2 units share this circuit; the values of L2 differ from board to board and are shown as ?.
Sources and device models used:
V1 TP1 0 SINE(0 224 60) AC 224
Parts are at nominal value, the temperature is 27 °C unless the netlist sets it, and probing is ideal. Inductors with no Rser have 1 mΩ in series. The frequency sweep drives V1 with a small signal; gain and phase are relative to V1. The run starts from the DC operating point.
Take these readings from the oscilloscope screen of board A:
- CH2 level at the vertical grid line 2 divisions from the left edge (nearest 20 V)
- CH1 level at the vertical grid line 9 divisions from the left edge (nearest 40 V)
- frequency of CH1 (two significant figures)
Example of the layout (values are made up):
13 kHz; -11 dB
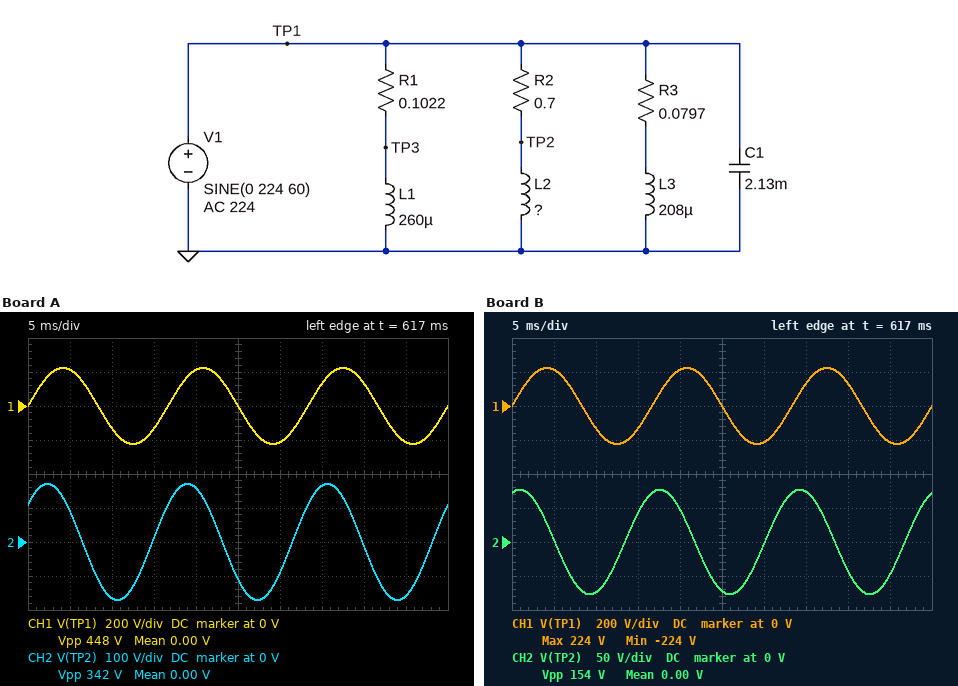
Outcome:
-160 V; -200 V; 60 Hz
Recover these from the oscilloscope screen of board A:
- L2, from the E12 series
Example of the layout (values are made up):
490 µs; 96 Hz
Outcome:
2.2 mH
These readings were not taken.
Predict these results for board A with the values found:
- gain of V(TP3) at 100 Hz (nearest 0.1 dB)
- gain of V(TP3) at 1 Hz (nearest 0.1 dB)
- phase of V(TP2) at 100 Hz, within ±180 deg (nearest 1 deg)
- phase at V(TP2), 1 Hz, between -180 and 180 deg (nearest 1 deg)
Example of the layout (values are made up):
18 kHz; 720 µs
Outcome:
-1.5 dB; -34.6 dB; 27 deg; 85 deg
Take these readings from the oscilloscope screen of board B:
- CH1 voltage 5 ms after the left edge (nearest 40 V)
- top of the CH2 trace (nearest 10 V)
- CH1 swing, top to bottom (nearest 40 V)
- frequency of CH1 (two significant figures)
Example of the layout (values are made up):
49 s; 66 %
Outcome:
200 V; 80 V; 440 V; 60 Hz
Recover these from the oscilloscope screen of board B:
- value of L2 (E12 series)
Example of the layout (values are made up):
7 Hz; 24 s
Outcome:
680 µH
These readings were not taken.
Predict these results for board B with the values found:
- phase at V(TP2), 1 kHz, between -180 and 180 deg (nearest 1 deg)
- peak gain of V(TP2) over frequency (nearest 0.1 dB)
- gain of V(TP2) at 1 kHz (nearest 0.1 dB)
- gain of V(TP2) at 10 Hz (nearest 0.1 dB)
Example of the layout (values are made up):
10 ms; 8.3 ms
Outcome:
9 deg; 0 dB; -0.1 dB; -24.3 dB
